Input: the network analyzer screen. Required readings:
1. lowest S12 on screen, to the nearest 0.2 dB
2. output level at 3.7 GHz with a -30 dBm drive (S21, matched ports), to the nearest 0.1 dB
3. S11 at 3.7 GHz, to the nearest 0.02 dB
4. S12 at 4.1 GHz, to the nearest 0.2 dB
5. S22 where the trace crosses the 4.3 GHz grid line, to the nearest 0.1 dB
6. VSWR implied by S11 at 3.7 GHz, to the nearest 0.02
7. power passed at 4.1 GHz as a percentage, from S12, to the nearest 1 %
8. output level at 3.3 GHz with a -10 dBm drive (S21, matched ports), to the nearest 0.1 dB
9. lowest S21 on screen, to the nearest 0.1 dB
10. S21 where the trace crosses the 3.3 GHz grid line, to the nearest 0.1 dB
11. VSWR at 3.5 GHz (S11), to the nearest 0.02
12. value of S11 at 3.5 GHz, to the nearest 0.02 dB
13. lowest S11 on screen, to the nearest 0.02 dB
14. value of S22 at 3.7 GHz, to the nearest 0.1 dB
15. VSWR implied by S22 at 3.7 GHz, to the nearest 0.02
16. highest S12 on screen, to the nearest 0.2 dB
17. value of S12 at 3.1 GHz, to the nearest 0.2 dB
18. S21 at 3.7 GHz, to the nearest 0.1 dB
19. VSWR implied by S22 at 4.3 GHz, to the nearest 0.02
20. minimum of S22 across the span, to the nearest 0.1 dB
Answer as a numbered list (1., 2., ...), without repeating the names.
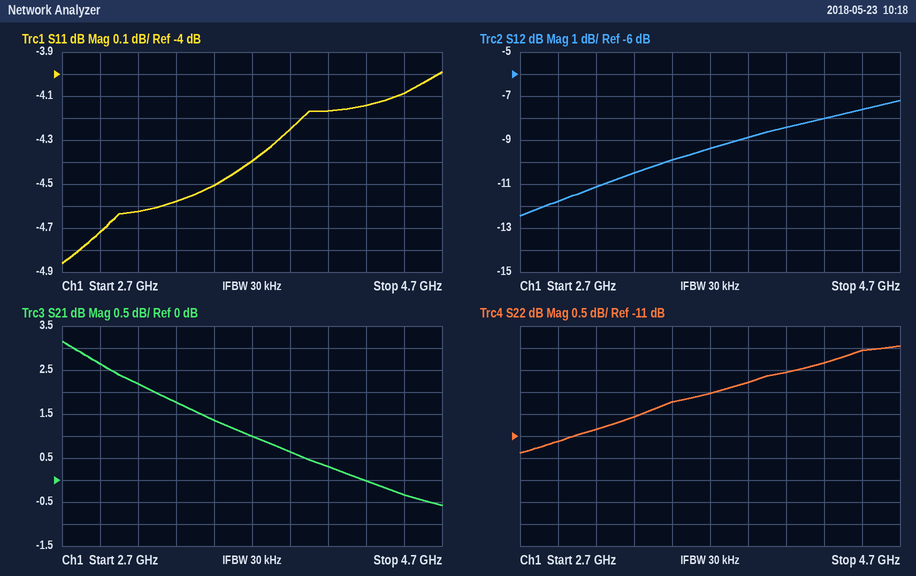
1. -12.4 dB
2. -29.0 dBm
3. -4.40 dB
4. -8.4 dB
5. -9.3 dB
6. 4.04
7. 14 %
8. -8.2 dBm
9. -0.6 dB
10. 1.8 dB
11. 3.94
12. -4.50 dB
13. -4.86 dB
14. -10.0 dB
15. 1.92
16. -7.2 dB
17. -11.2 dB
18. 1.0 dB
19. 2.04
20. -11.4 dB
